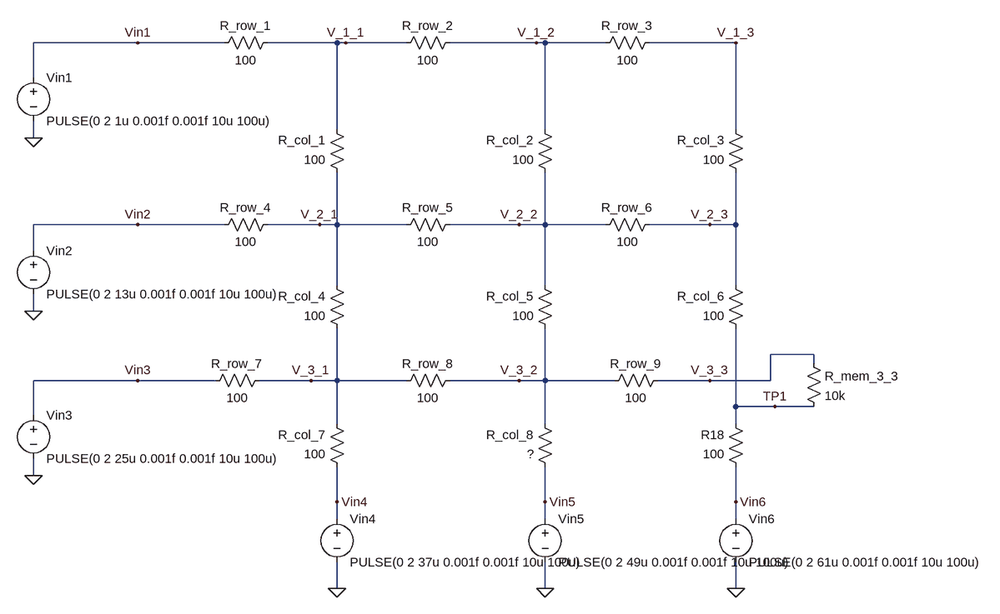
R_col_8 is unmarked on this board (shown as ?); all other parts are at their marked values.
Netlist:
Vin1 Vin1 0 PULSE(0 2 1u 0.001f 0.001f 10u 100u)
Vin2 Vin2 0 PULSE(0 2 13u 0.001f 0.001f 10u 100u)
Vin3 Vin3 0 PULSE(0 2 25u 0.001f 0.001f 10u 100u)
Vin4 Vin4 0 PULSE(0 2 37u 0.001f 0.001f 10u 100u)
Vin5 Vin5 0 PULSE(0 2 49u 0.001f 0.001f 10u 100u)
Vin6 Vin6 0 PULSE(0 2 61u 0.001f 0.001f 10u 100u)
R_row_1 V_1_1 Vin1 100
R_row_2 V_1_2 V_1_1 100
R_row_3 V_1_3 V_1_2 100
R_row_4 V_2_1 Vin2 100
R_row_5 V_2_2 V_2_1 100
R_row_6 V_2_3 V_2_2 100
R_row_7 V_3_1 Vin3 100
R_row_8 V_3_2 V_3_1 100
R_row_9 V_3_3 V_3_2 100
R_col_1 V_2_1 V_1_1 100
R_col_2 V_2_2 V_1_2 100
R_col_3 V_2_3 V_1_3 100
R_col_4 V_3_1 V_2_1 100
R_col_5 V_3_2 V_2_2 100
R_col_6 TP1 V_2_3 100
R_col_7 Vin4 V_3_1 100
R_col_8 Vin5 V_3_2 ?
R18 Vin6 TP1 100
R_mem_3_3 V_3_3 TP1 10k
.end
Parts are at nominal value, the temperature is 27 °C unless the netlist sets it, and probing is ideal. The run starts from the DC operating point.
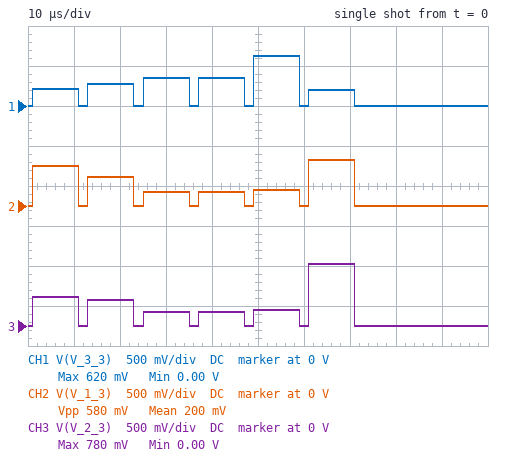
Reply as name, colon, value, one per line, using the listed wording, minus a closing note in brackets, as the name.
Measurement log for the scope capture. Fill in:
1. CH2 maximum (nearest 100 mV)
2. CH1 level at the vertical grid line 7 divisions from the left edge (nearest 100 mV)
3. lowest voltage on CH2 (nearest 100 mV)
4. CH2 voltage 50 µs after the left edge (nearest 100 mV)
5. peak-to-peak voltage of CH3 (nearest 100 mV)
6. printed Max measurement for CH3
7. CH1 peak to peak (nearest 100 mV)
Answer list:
CH2 maximum: 600 mV
CH1 level at the vertical grid line 7 divisions from the left edge: 200 mV
lowest voltage on CH2: 0 V
CH2 voltage 50 µs after the left edge: 200 mV
peak-to-peak voltage of CH3: 800 mV
printed Max measurement for CH3: 780 mV
CH1 peak to peak: 600 mV
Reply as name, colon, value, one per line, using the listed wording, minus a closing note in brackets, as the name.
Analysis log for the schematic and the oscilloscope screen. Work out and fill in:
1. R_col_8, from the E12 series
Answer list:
R_col_8, from the E12 series: 180 Ω
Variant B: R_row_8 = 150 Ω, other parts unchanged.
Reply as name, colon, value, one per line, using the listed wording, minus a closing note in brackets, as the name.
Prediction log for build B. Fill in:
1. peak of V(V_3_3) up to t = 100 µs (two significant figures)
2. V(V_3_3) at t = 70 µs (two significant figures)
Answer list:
peak of V(V_3_3) up to t = 100 µs: 690 mV
V(V_3_3) at t = 70 µs: 210 mV
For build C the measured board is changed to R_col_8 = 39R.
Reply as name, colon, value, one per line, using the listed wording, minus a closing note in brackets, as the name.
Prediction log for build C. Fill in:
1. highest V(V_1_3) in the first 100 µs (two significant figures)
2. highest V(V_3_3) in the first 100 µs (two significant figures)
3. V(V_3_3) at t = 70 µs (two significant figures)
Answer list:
highest V(V_1_3) in the first 100 µs: 550 mV
highest V(V_3_3) in the first 100 µs: 1.3 V
V(V_3_3) at t = 70 µs: 100 mV
